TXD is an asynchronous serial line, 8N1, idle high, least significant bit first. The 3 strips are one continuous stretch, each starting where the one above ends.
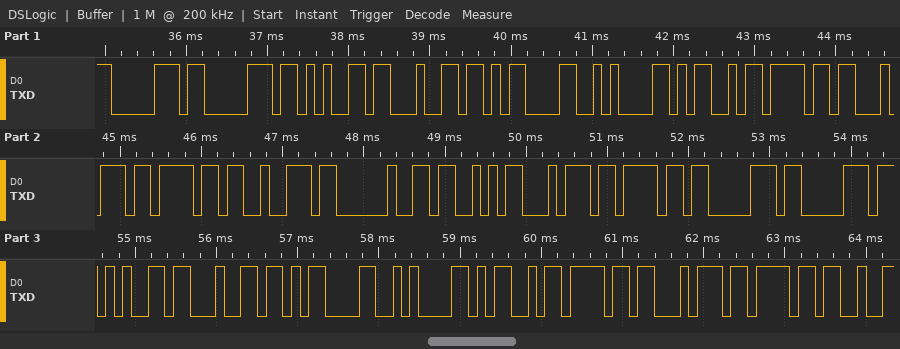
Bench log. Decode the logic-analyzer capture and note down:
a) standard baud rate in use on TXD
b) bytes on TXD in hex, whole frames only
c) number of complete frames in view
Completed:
9600 baud
70 70 65 64 0D 0A 4D 6F 74 6F 72 20 53 74 6F 70 70 65 64 0D 0A 4D 6F 74 6F
25
